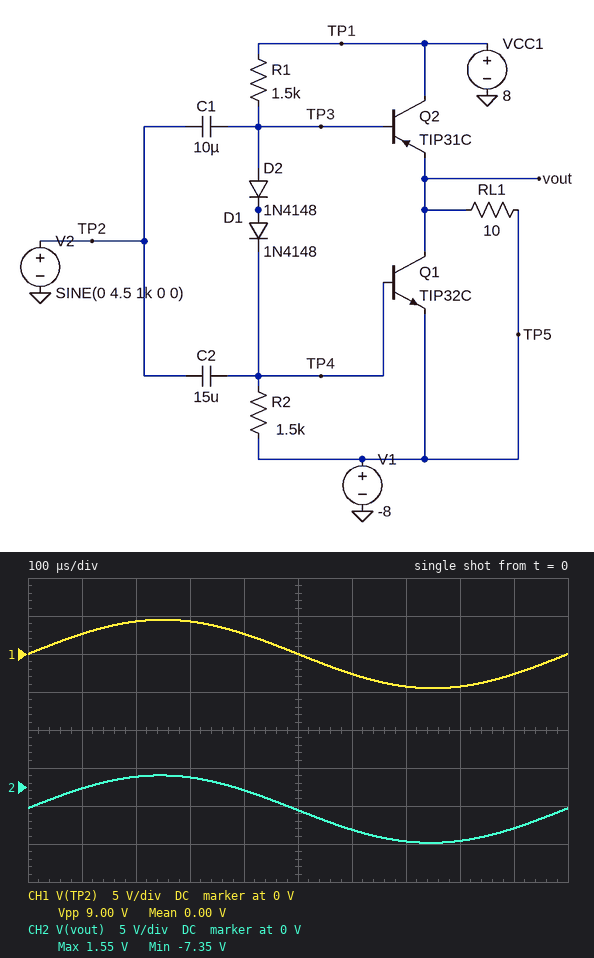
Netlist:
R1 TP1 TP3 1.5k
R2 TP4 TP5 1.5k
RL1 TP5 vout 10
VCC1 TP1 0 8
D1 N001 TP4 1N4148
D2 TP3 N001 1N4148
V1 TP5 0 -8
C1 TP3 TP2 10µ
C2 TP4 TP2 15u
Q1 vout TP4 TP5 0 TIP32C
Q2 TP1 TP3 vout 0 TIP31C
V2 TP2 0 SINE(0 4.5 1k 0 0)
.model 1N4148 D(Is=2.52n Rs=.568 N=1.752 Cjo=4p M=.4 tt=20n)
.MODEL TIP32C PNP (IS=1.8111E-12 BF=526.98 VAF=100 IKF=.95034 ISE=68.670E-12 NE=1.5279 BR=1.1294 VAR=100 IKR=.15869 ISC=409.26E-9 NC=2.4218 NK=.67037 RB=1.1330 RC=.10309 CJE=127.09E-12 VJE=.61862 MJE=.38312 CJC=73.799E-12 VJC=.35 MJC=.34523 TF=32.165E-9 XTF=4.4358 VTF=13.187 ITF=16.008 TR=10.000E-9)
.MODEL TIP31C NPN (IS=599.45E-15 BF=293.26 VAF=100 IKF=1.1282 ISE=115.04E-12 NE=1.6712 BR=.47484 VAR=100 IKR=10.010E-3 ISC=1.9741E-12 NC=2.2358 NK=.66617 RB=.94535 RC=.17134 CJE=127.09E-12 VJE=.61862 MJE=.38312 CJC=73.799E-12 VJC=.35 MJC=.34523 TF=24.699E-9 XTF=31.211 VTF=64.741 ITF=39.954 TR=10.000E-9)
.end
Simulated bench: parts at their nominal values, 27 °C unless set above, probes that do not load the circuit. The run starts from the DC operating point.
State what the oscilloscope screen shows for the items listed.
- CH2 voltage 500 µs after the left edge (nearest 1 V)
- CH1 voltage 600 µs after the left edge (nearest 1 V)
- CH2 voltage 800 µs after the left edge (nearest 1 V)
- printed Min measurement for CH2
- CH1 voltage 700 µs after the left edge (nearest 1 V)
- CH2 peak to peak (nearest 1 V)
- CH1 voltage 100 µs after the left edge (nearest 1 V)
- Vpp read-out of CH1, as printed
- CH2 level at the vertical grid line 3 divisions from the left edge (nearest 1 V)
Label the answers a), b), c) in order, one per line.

a) -3 V
b) -3 V
c) -7 V
d) -7.35 V
e) -4 V
f) 9 V
g) 3 V
h) 9.00 V
i) 1 V
